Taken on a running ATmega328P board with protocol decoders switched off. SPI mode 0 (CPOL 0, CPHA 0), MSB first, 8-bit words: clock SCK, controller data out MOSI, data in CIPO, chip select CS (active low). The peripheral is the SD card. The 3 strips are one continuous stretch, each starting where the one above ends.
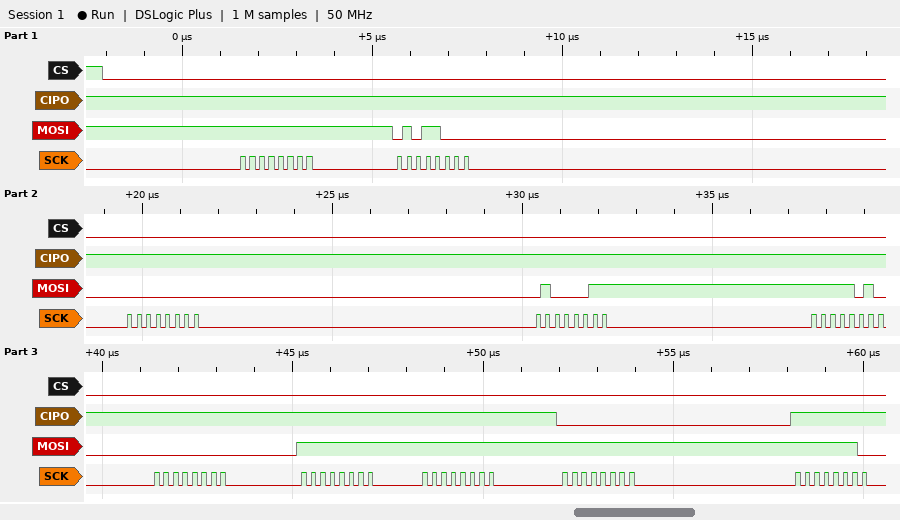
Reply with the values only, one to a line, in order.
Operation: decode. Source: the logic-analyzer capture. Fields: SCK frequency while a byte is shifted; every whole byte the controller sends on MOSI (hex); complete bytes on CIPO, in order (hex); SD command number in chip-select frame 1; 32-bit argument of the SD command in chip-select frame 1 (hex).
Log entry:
4 MHz
0xFF 0x58 0x00 0x43 0xFA 0x00 0xFF 0xFF 0xFF 0xFE
0xFF 0xFF 0xFF 0xFF 0xFF 0xFF 0xFF 0xFF 0x00 0xFF
CMD24
0x0043FA00
